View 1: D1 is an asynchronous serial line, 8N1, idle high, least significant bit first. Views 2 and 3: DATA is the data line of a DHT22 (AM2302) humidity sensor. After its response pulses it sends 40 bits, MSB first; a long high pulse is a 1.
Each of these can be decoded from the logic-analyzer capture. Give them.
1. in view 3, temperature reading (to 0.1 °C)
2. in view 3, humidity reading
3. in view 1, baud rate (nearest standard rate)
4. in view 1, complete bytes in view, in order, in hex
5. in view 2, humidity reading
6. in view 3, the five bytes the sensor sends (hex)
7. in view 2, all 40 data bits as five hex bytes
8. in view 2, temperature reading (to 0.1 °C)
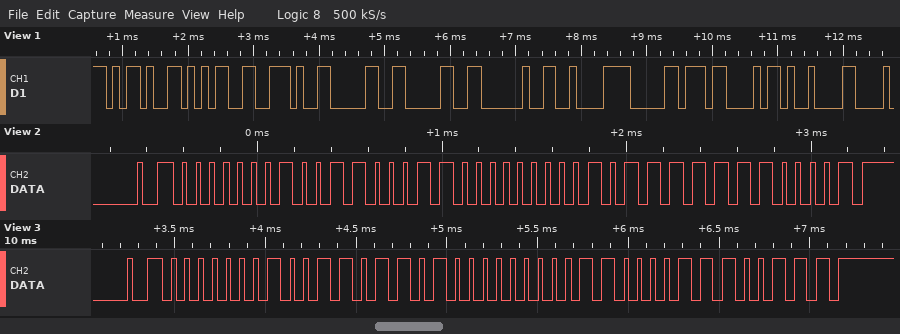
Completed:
-4.8 °C
31.0 %
9600 baud
0x2D 0x35 0x2E 0x30 0x30 0x20 0xC2 0xB0 0x43 0x09
30.5 %
01 36 80 30 E7
01 31 80 2F E1
-4.7 °C
